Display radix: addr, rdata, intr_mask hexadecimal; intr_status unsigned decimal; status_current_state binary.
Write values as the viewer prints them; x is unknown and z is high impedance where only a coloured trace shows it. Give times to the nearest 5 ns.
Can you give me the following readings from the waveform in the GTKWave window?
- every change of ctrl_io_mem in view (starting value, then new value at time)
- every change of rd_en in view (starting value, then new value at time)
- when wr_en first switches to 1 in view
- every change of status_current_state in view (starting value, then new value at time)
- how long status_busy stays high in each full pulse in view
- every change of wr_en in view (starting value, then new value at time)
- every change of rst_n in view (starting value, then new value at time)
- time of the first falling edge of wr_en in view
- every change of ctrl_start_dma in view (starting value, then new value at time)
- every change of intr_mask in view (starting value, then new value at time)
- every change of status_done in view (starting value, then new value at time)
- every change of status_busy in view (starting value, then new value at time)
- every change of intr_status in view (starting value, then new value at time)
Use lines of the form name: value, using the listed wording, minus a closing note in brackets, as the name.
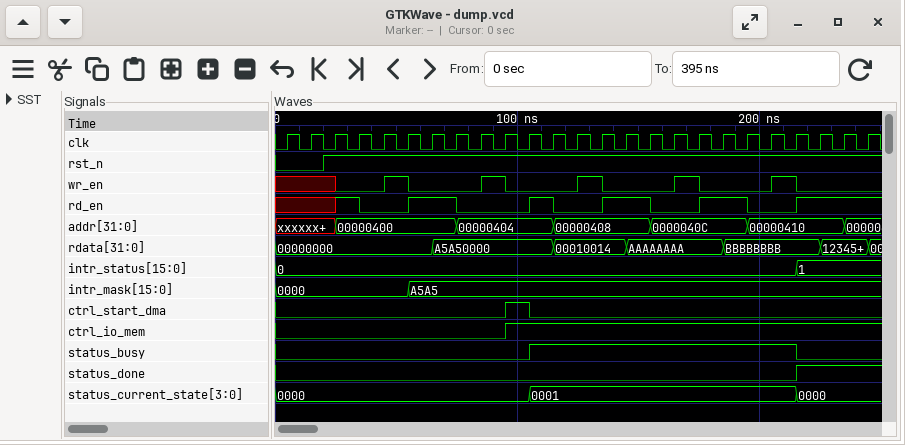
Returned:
every change of ctrl_io_mem in view: 0, 1 at 95 ns
every change of rd_en in view: x, 1 at 25 ns, 0 at 35 ns, 1 at 55 ns, 0 at 75 ns, 1 at 105 ns, 0 at 115 ns, 1 at 135 ns, 0 at 155 ns, 1 at 175 ns, 0 at 195 ns, 1 at 215 ns
when wr_en first switches to 1 in view: 45 ns
every change of status_current_state in view: 0000, 0001 at 105 ns, 0000 at 215 ns
how long status_busy stays high in each full pulse in view: 110 ns
every change of wr_en in view: x, 0 at 25 ns, 1 at 45 ns, 0 at 55 ns, 1 at 85 ns, 0 at 95 ns, 1 at 125 ns, 0 at 135 ns, 1 at 165 ns, 0 at 175 ns, 1 at 205 ns, 0 at 215 ns
every change of rst_n in view: 0, 1 at 20 ns
time of the first falling edge of wr_en in view: 55 ns
every change of ctrl_start_dma in view: 0, 1 at 95 ns, 0 at 105 ns
every change of intr_mask in view: 0000, A5A5 at 55 ns
every change of status_done in view: 0, 1 at 215 ns
every change of status_busy in view: 0, 1 at 105 ns, 0 at 215 ns
every change of intr_status in view: 0, 1 at 215 ns
